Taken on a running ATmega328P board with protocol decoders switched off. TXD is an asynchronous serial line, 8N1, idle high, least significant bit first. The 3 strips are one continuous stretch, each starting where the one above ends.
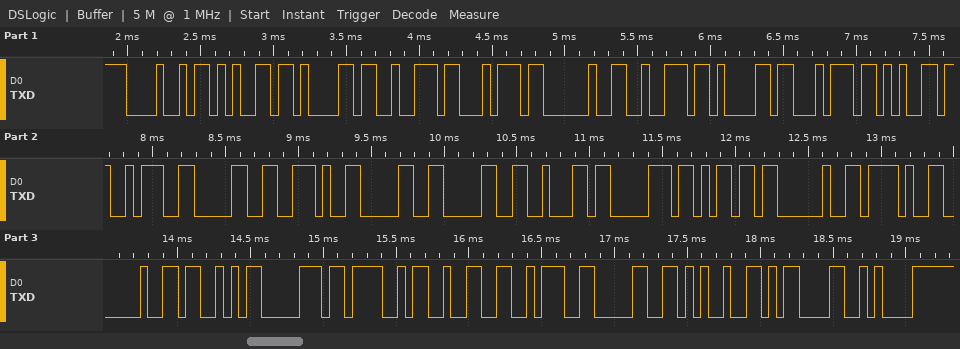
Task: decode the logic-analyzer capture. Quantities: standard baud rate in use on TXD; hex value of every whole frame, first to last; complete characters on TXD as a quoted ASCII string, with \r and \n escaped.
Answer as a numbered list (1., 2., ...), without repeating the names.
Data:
1. 19200 baud
2. 0x48 0x65 0x61 0x72 0x74 0x20 0x72 0x61 0x74 0x65 0x3A 0x30 0x2E 0x30 0x30 0x62 0x70 0x6D 0x20 0x2F 0x20 0x53 0x70 0x4F 0x32 0x3A 0x30 0x25 0x0D 0x0A
3. "Heart rate:0.00bpm / SpO2:0%\r\n"
